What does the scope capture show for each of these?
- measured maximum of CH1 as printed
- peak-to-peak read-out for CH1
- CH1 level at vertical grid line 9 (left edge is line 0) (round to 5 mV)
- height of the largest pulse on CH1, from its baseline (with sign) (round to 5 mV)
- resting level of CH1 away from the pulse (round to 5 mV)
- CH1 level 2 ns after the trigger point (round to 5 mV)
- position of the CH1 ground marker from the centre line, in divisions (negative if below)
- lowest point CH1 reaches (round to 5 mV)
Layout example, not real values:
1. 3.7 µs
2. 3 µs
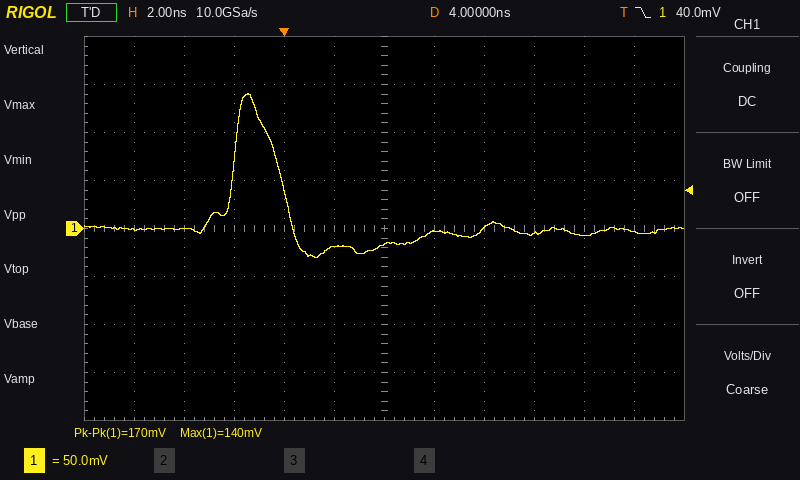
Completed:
1. 140 mV
2. 170 mV
3. -5 mV
4. +140 mV
5. 0 mV
6. -20 mV
7. 0.0 div
8. -30 mV
